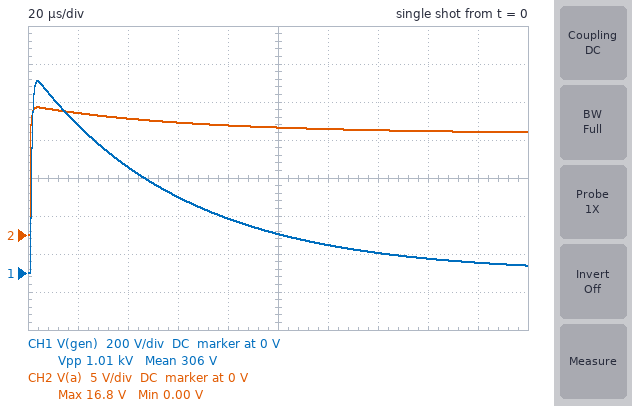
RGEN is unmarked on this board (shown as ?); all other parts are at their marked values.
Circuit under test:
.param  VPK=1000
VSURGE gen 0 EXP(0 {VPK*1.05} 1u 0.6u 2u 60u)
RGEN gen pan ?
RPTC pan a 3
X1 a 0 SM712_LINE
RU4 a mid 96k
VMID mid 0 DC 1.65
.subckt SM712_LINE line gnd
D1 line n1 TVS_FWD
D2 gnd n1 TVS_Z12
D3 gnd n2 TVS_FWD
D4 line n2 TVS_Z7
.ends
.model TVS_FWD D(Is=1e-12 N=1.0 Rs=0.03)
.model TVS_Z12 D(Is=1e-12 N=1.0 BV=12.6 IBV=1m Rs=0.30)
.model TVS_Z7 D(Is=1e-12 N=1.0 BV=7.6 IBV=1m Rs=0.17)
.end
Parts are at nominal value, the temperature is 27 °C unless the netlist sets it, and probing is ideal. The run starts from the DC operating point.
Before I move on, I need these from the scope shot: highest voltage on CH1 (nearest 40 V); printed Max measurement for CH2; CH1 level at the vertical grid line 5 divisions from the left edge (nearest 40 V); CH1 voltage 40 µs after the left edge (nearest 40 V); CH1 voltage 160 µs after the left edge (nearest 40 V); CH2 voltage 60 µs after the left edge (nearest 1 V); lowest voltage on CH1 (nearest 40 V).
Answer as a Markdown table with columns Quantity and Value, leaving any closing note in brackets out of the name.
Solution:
| Quantity | Value |
|---|---|
| highest voltage on CH1 | 1.00 kV |
| printed Max measurement for CH2 | 16.8 V |
| CH1 level at the vertical grid line 5 divisions from the left edge | 200 V |
| CH1 voltage 40 µs after the left edge | 560 V |
| CH1 voltage 160 µs after the left edge | 80 V |
| CH2 voltage 60 µs after the left edge | 15 V |
| lowest voltage on CH1 | 0 V |
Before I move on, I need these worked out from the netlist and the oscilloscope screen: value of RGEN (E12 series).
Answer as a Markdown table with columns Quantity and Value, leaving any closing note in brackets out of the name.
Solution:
| Quantity | Value |
|---|---|
| value of RGEN | 100 Ω |
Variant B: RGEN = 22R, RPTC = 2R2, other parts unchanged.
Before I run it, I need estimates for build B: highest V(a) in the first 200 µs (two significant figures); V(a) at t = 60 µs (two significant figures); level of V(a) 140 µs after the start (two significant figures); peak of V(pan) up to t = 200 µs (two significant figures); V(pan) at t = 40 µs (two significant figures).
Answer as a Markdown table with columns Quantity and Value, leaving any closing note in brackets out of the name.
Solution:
| Quantity | Value |
|---|---|
| highest V(a) in the first 200 µs | 27 V |
| V(a) at t = 60 µs | 19 V |
| level of V(a) 140 µs after the start | 15 V |
| peak of V(pan) up to t = 200 µs | 120 V |
| V(pan) at t = 40 µs | 70 V |
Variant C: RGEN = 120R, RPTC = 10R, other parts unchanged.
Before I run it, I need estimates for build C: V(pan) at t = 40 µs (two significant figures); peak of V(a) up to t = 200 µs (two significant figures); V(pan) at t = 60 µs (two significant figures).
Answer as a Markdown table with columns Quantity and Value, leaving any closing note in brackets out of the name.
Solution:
| Quantity | Value |
|---|---|
| V(pan) at t = 40 µs | 57 V |
| peak of V(a) up to t = 200 µs | 16 V |
| V(pan) at t = 60 µs | 44 V |
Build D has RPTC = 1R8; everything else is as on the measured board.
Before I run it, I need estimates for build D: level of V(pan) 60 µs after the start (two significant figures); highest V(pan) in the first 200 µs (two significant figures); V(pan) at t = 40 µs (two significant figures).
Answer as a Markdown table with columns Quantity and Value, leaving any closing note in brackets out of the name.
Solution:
| Quantity | Value |
|---|---|
| level of V(pan) 60 µs after the start | 22 V |
| highest V(pan) in the first 200 µs | 34 V |
| V(pan) at t = 40 µs | 25 V |
